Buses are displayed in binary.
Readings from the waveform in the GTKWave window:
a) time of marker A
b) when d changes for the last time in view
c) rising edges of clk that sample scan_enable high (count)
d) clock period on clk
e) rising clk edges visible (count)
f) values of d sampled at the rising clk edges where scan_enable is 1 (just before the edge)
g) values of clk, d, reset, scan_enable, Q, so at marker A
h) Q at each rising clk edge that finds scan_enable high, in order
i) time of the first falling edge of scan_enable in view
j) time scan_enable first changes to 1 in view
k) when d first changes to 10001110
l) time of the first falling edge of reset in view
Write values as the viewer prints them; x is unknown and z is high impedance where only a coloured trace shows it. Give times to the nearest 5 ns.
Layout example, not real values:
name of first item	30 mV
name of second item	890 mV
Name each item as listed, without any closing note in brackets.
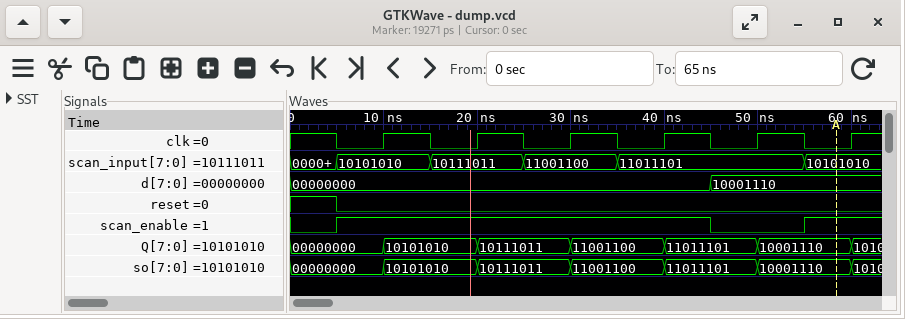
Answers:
time of marker A	60 ns
when d changes for the last time in view	45 ns
rising edges of clk that sample scan_enable high	5
clock period on clk	10 ns
rising clk edges visible	6
values of d sampled at the rising clk edges where scan_enable is 1	00000000, 00000000, 00000000, 00000000, 10001110
values of clk, d, reset, scan_enable, Q, so at marker A	clk=0, d=10001110, reset=0, scan_enable=1, Q=10001110, so=10001110
Q at each rising clk edge that finds scan_enable high, in order	00000000, 10101010, 10111011, 11001100, 10001110
time of the first falling edge of scan_enable in view	45 ns
time scan_enable first changes to 1 in view	5 ns
when d first changes to 10001110	45 ns
time of the first falling edge of reset in view	5 ns
